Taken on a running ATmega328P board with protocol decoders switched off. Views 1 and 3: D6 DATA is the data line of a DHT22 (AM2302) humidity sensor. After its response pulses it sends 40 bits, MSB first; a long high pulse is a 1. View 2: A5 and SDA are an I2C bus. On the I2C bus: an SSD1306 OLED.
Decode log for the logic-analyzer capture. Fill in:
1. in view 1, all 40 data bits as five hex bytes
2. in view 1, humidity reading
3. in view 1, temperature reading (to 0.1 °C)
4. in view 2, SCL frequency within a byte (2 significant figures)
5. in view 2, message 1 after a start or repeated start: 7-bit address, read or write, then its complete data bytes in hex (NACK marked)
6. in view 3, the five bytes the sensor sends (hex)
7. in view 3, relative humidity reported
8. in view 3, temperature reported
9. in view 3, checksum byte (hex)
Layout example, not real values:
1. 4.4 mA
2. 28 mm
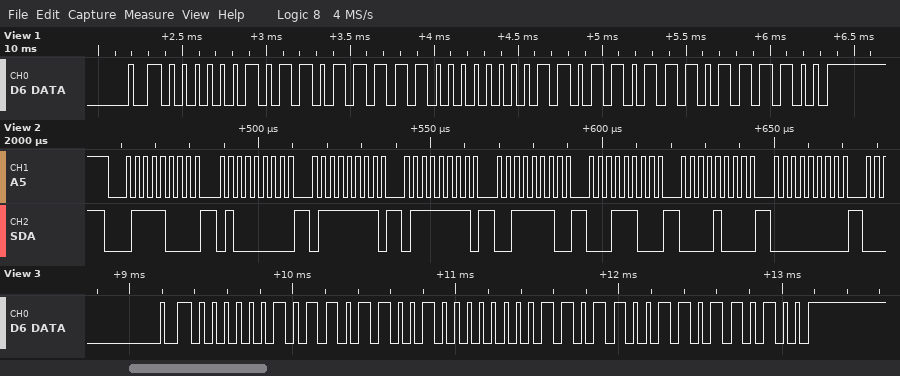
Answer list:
1. 02 DF 00 DB BC
2. 73.5 %
3. 21.9 °C
4. 400 kHz
5. 0x3C write: 40 7F 7F 3E 1C 08 00
6. 02 D9 00 D9 B4
7. 72.9 %
8. 21.7 °C
9. 0xB4
